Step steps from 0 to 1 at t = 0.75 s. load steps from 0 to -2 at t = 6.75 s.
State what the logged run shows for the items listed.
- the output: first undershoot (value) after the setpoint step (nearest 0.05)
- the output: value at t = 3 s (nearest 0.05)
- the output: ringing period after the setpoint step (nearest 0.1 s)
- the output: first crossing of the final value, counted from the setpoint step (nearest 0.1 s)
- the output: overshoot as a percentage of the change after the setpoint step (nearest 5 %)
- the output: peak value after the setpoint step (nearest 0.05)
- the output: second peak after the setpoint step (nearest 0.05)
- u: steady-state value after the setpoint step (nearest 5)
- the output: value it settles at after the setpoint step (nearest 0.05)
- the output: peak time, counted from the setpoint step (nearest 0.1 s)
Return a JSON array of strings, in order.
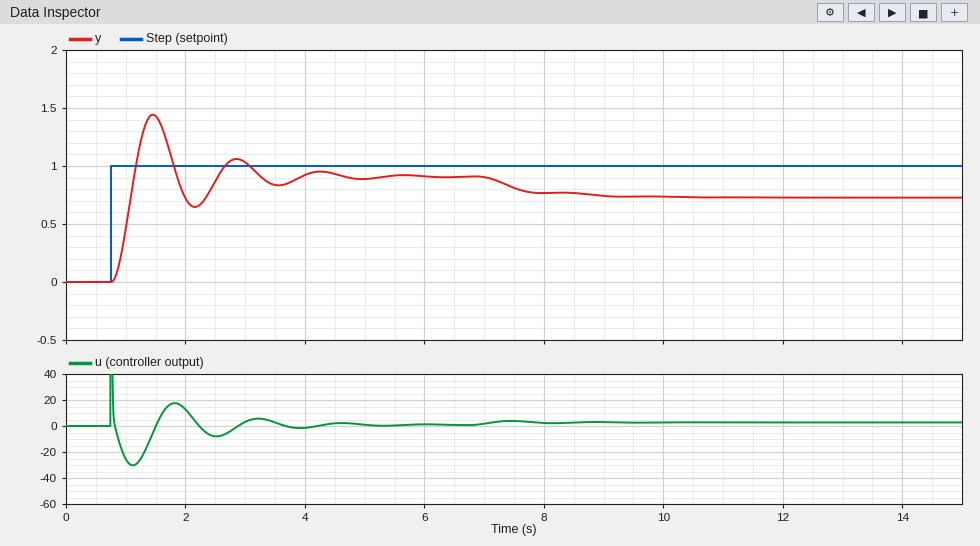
["0.65", "1.05", "1.4 s", "0.4 s", "60 %", "1.45", "1.05", "0", "0.90", "0.7 s"]
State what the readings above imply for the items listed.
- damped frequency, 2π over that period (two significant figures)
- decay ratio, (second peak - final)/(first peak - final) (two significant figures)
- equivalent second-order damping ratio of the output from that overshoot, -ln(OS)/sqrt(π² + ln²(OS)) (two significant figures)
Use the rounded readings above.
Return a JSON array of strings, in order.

["4.5 rad/s", "0.27", "0.16"]
